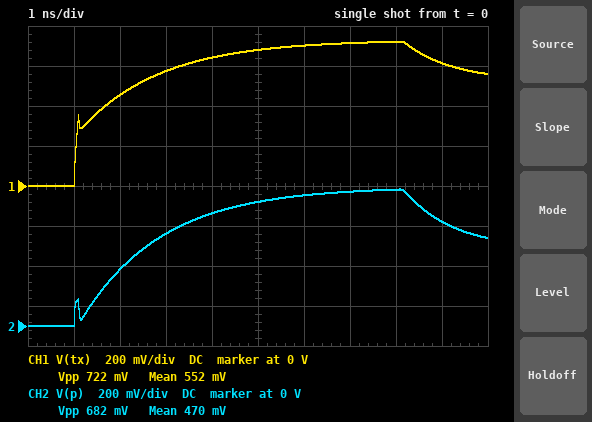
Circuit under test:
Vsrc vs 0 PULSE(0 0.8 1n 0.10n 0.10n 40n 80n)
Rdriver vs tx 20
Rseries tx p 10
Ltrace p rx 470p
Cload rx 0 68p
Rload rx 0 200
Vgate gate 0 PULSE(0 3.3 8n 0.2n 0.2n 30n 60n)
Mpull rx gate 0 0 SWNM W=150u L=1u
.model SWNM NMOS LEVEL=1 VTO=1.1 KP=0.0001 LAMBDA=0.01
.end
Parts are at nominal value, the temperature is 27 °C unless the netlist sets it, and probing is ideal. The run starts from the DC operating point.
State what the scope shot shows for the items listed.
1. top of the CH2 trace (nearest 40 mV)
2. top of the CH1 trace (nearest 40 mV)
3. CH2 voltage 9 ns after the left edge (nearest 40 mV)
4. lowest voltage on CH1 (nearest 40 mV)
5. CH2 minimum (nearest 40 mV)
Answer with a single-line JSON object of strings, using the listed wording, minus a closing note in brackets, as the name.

{"top of the CH2 trace": "680 mV", "top of the CH1 trace": "720 mV", "CH2 voltage 9 ns after the left edge": "520 mV", "lowest voltage on CH1": "0 V", "CH2 minimum": "0 V"}
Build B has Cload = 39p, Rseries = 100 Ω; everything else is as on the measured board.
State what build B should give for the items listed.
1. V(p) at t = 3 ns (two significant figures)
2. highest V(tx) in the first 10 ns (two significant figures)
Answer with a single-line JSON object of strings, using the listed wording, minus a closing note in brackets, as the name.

{"V(p) at t = 3 ns": "240 mV", "highest V(tx) in the first 10 ns": "740 mV"}
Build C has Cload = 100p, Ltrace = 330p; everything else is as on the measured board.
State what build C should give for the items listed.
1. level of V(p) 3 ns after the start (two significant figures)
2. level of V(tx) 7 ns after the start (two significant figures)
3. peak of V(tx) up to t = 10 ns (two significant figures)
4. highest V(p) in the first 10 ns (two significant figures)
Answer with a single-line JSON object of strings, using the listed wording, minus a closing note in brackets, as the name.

{"level of V(p) 3 ns after the start": "360 mV", "level of V(tx) 7 ns after the start": "680 mV", "peak of V(tx) up to t = 10 ns": "700 mV", "highest V(p) in the first 10 ns": "650 mV"}
